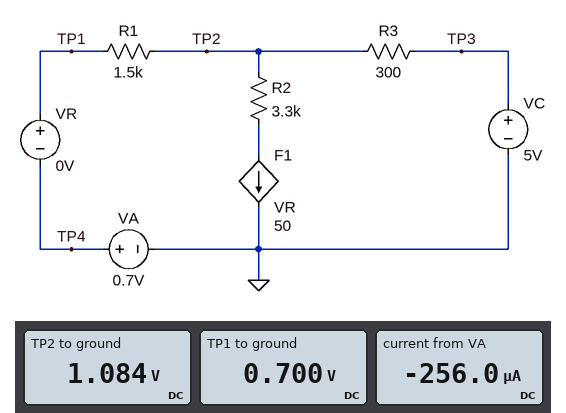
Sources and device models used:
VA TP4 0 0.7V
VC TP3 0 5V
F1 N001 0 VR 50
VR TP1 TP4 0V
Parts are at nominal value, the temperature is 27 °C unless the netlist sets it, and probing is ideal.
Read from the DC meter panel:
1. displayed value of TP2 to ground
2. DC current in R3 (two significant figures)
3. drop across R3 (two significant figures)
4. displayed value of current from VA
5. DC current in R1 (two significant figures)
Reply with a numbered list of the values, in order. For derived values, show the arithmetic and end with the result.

1. 1.084 V
2. (5 V - 1.084 V) / 300 Ω = 13 mA
3. 5 V - 1.084 V = 3.9 V
4. -256.0 µA
5. (1.084 V - 700 mV) / 1.5 kΩ = 260 µA
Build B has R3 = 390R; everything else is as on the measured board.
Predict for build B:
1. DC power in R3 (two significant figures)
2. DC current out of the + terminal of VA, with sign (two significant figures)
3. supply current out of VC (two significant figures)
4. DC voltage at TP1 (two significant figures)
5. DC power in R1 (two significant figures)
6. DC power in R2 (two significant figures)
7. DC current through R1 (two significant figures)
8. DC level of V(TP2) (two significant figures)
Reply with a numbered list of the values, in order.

1. 41 mW
2. -200 µA
3. 10 mA
4. 700 mV
5. 61 µW
6. 330 mW
7. 200 µA
8. 1.0 V
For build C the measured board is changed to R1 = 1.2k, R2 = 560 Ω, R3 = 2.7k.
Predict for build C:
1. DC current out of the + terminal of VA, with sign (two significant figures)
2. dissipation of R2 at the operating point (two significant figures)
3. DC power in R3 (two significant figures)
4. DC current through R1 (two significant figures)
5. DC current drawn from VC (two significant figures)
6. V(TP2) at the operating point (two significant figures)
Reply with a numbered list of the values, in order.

1. -31 µA
2. 1.3 mW
3. 6.7 mW
4. 31 µA
5. 1.6 mA
6. 740 mV
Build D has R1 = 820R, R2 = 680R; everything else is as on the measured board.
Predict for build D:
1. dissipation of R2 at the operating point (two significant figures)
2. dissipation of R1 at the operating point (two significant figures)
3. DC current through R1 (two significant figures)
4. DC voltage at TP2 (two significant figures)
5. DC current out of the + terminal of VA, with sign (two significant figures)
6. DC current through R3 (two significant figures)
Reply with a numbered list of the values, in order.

1. 120 mW
2. 58 µW
3. 270 µA
4. 920 mV
5. -270 µA
6. 14 mA
